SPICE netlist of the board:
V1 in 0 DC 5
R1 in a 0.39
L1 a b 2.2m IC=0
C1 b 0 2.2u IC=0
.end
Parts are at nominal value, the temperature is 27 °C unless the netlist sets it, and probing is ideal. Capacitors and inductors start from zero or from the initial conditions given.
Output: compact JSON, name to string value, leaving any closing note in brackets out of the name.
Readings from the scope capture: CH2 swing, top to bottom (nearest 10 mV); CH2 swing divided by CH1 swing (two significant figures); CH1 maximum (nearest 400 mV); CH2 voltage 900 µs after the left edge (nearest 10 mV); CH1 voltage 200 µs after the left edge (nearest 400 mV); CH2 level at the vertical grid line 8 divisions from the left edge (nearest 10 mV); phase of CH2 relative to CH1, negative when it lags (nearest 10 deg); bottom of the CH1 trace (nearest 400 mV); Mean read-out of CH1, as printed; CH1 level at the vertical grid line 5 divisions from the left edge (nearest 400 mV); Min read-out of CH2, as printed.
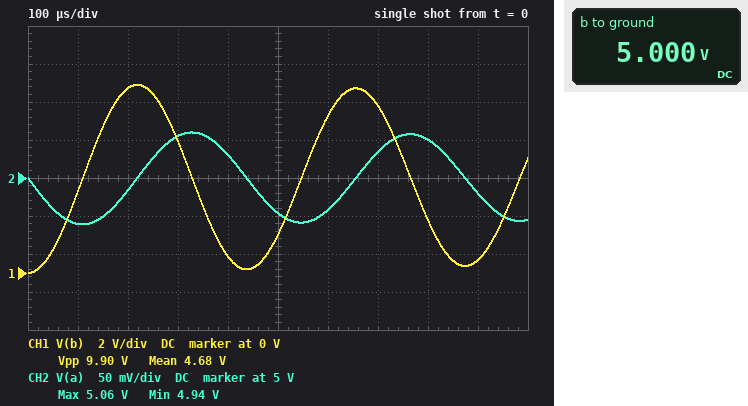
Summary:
{"CH2 swing, top to bottom": "120 mV", "CH2 swing divided by CH1 swing": "0.012", "CH1 maximum": "10.0 V", "CH2 voltage 900 µs after the left edge": "4.98 V", "CH1 voltage 200 µs after the left edge": "9.6 V", "CH2 level at the vertical grid line 8 divisions from the left edge": "5.05 V", "phase of CH2 relative to CH1, negative when it lags": "-90 deg", "bottom of the CH1 trace": "0 V", "Mean read-out of CH1, as printed": "4.68 V", "CH1 level at the vertical grid line 5 divisions from the left edge": "2.0 V", "Min read-out of CH2, as printed": "4.94 V"}
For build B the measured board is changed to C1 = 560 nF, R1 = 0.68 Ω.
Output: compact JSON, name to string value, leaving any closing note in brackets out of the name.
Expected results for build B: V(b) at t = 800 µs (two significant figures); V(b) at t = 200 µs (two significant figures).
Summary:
{"V(b) at t = 800 µs": "8.1 V", "V(b) at t = 200 µs": "970 mV"}
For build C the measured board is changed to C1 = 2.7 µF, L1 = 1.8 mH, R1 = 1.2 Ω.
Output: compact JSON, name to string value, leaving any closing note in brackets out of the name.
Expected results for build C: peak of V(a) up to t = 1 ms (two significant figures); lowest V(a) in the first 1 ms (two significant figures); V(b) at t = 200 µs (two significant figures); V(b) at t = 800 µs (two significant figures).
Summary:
{"peak of V(a) up to t = 1 ms": "5.2 V", "lowest V(a) in the first 1 ms": "4.8 V", "V(b) at t = 200 µs": "9.5 V", "V(b) at t = 800 µs": "3.3 V"}
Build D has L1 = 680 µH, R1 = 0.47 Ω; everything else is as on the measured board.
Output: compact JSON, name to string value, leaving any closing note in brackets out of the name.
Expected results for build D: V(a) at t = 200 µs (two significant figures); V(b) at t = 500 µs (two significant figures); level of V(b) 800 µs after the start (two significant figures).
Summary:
{"V(a) at t = 200 µs": "5.1 V", "V(b) at t = 500 µs": "1.0 V", "level of V(b) 800 µs after the start": "5.9 V"}
